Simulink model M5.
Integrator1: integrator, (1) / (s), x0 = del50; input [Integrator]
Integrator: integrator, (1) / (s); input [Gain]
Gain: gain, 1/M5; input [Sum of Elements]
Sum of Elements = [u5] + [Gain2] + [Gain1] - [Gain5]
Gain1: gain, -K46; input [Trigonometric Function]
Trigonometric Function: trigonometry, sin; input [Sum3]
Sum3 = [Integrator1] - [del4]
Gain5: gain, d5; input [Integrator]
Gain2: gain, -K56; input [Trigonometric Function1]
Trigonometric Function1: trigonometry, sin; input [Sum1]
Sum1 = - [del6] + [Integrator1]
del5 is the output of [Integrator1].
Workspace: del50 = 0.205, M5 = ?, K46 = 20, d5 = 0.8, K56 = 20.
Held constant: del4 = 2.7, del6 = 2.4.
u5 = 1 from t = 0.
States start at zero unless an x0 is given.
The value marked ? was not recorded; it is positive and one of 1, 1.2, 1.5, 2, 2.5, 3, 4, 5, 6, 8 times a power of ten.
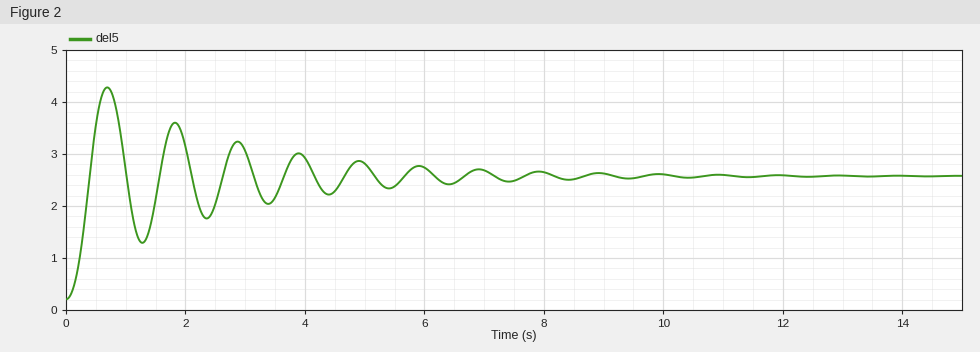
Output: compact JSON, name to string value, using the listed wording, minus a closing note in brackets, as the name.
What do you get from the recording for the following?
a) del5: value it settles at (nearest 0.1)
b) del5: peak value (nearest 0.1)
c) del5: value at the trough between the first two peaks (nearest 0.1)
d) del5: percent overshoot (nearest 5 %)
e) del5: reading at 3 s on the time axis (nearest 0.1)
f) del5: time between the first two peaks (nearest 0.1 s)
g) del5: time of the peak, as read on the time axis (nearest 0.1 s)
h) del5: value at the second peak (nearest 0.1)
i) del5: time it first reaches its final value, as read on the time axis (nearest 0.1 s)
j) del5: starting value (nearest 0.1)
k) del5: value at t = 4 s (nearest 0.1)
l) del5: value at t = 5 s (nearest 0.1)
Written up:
{"del5: value it settles at": "2.6", "del5: peak value": "4.3", "del5: value at the trough between the first two peaks": "1.3", "del5: percent overshoot": "70 %", "del5: reading at 3 s on the time axis": "3.1", "del5: time between the first two peaks": "1.1 s", "del5: time of the peak, as read on the time axis": "0.7 s", "del5: value at the second peak": "3.6", "del5: time it first reaches its final value, as read on the time axis": "0.4 s", "del5: starting value": "0.2", "del5: value at t = 4 s": "2.9", "del5: value at t = 5 s": "2.8"}
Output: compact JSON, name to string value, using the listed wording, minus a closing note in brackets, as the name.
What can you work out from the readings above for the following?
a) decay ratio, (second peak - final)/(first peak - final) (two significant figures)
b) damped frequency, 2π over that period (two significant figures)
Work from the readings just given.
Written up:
{"decay ratio, (second peak - final)/(first peak - final)": "0.59", "damped frequency, 2π over that period": "5.7 rad/s"}
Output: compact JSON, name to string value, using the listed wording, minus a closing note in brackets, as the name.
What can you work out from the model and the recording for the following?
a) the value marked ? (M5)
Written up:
{"the value marked ?": "1"}
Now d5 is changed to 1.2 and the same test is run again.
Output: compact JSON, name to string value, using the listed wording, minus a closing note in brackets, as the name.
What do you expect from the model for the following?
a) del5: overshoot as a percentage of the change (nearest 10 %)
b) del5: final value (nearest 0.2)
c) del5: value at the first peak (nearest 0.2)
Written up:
{"del5: overshoot as a percentage of the change": "60 %", "del5: final value": "2.6", "del5: value at the first peak": "4.0"}
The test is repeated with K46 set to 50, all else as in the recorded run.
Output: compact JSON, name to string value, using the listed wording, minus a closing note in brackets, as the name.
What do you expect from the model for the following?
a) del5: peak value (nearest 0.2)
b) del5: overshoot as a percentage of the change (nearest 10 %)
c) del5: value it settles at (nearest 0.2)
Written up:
{"del5: peak value": "4.4", "del5: overshoot as a percentage of the change": "80 %", "del5: value it settles at": "2.6"}
